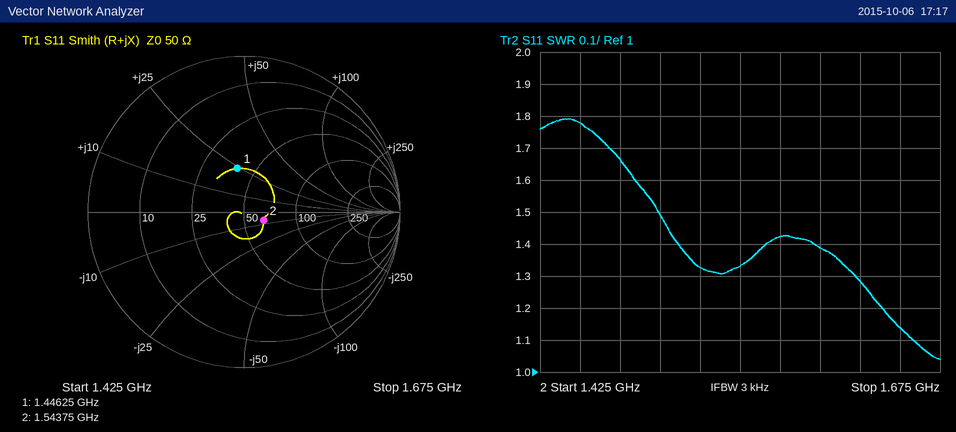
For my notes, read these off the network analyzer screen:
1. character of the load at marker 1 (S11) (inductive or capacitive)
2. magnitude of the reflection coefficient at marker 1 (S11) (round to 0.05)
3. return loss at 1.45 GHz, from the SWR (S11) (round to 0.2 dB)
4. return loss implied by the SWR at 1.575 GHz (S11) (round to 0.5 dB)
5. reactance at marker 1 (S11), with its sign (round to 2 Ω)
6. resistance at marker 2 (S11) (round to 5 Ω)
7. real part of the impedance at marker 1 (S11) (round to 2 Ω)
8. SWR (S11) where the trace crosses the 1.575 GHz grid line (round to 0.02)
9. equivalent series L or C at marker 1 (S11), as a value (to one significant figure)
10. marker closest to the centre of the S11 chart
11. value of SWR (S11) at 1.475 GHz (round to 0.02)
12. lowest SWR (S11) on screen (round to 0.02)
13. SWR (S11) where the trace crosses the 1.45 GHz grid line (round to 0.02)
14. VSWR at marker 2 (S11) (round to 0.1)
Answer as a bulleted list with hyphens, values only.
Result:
- inductive
- 0.30
- 11.0 dB
- 15.0 dB
- +24 Ω
- 65 Ω
- 40 Ω
- 1.42
- 3 nH
- marker 2
- 1.66
- 1.04
- 1.78
- 1.3
